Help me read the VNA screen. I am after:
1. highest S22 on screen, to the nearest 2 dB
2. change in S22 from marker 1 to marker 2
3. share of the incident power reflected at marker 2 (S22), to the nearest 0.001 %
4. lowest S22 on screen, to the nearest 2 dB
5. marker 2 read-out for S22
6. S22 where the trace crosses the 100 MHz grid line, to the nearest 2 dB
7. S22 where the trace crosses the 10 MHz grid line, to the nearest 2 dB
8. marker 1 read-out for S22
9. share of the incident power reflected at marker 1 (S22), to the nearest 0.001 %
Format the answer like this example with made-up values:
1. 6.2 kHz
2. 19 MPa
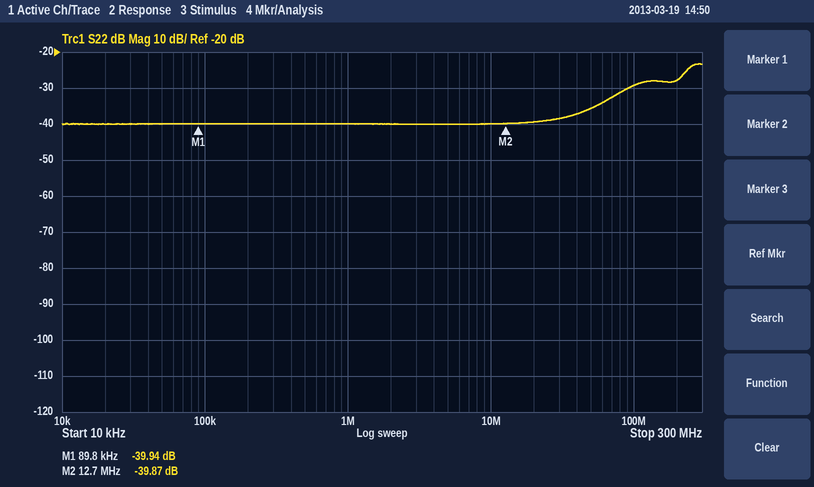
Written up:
1. -24 dB
2. 0.07 dB
3. 0.010 %
4. -40 dB
5. -39.87 dB
6. -30 dB
7. -40 dB
8. -39.94 dB
9. 0.010 %
